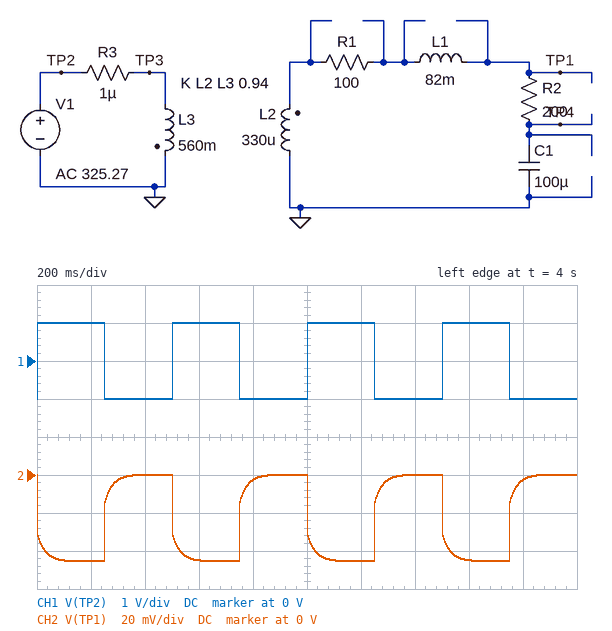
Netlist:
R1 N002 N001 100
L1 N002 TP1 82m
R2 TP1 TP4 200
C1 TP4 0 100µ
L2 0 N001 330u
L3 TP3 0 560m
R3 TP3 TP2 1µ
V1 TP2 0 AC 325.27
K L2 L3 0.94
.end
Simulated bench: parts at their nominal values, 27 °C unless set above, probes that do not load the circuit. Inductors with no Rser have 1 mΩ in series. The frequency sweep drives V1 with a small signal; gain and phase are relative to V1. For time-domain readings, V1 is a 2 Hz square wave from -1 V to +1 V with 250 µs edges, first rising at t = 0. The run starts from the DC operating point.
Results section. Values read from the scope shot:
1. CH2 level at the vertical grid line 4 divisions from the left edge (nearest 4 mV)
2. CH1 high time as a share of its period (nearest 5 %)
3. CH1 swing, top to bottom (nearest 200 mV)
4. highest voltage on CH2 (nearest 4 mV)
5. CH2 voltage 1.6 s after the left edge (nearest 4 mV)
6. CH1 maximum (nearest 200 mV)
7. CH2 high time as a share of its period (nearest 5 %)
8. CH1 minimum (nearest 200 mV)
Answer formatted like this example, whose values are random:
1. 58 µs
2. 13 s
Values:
1. -4 mV
2. 50 %
3. 2.0 V
4. 0 V
5. -44 mV
6. 1.0 V
7. 50 %
8. -1.0 V
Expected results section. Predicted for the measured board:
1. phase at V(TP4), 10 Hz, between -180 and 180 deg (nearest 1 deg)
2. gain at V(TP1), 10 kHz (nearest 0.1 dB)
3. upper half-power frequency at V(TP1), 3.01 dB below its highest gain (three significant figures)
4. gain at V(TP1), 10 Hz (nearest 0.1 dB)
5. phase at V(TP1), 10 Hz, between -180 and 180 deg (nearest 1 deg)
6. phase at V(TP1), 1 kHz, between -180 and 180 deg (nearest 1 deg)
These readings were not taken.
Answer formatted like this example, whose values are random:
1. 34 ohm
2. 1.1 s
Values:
1. 117 deg
2. -61.1 dB
3. 17.3 Hz
4. -35.2 dB
5. 169 deg
6. 120 deg
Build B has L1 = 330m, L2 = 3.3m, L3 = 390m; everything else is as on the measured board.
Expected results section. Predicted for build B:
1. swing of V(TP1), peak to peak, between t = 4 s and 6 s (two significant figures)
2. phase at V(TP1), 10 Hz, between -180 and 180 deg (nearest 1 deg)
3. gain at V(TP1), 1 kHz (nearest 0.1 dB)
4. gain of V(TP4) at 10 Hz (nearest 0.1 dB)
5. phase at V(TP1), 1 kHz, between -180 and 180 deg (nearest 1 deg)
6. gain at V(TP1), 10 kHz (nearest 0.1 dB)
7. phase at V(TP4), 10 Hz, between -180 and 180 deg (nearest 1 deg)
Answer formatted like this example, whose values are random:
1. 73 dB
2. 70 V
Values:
1. 170 mV
2. 166 deg
3. -41.7 dB
4. -27.6 dB
5. 98 deg
6. -61.6 dB
7. 115 deg
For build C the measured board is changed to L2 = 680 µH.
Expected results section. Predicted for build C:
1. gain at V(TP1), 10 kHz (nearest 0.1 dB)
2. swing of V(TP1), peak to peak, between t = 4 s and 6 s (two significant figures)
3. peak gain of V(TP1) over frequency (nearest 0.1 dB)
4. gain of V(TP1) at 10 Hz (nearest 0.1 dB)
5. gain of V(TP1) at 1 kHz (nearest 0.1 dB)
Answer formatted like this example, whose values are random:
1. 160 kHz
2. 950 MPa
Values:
1. -57.9 dB
2. 66 mV
3. -29.7 dB
4. -32.1 dB
5. -39.2 dB
